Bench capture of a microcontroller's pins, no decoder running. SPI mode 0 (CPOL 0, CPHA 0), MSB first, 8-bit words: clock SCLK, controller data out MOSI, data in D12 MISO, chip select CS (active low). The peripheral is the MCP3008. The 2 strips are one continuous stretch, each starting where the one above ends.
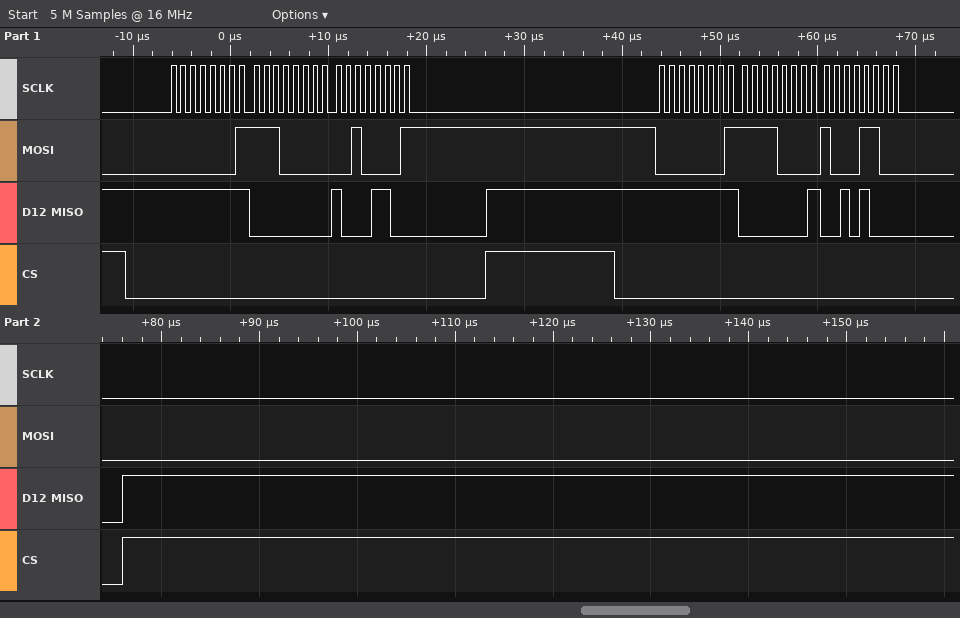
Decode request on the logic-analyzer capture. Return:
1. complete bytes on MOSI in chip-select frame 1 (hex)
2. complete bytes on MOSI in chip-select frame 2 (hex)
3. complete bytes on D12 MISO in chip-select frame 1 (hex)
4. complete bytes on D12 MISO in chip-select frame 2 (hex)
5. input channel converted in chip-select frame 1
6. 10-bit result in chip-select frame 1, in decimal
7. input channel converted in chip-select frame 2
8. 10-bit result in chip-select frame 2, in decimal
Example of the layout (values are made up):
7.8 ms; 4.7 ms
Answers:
01 E0 21; 01 F0 8C; FF 00 8C; FF 01 28; 6; 140; 7; 296
